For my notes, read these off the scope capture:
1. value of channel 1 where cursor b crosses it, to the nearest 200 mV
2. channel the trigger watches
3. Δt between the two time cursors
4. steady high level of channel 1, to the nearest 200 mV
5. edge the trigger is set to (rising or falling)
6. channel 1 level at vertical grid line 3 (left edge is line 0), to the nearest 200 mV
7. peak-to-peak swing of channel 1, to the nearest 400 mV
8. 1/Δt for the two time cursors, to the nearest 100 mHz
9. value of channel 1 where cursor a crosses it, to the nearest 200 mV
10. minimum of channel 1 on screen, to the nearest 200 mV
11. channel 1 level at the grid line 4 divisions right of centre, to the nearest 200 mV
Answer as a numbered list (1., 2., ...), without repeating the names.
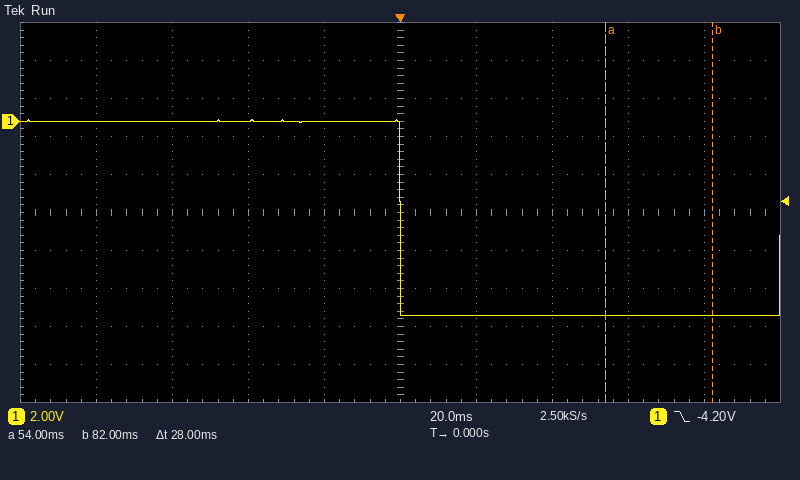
1. -10.2 V
2. channel 1
3. 28 ms
4. 0.0 V
5. falling
6. 0.0 V
7. 10.4 V
8. 35.7 Hz
9. -10.2 V
10. -10.2 V
11. -10.2 V
